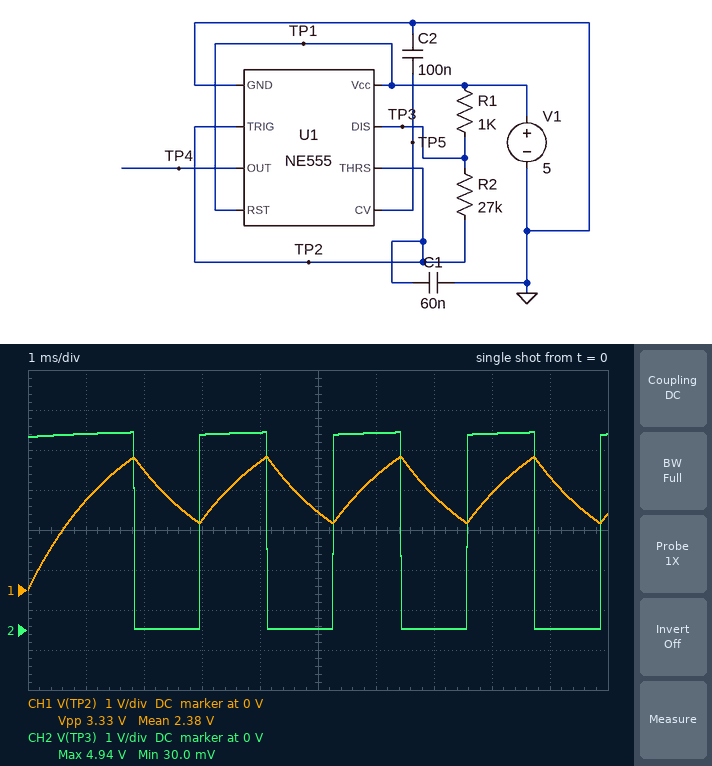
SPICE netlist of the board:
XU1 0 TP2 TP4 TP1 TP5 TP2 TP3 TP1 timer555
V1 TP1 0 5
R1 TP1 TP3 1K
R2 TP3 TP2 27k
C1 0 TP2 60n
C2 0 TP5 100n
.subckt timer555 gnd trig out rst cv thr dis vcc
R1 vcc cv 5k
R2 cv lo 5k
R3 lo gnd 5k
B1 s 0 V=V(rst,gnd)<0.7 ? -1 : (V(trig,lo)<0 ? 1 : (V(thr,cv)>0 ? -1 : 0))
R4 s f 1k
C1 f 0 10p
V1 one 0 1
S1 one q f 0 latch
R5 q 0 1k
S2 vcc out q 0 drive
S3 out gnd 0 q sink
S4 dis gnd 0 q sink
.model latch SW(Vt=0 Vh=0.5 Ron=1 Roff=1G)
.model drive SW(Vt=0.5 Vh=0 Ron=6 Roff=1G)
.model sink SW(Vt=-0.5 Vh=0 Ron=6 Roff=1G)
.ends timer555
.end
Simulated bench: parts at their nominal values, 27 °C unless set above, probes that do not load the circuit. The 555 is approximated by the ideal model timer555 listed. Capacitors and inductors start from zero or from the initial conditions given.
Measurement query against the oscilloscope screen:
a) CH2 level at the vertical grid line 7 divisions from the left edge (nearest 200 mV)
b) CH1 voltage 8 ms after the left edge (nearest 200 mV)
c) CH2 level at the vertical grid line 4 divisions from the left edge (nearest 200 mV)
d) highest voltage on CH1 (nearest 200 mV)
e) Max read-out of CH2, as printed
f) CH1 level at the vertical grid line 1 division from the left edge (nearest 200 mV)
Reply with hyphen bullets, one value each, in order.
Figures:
- 0 V
- 2.4 V
- 5.0 V
- 3.4 V
- 4.94 V
- 2.2 V
